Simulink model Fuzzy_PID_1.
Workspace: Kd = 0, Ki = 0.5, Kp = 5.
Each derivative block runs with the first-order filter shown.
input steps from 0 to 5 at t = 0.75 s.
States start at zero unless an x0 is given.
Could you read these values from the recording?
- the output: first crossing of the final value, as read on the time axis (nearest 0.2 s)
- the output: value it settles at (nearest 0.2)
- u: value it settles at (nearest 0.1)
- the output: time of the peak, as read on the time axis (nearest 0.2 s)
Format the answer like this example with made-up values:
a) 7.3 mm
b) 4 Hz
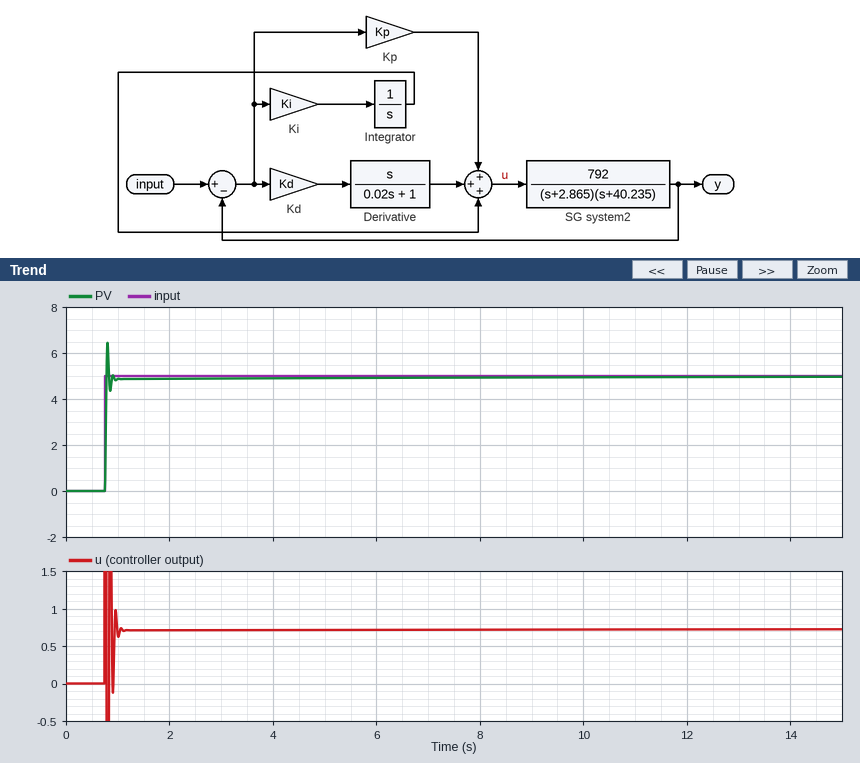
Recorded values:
a) 0.8 s
b) 5.0
c) 0.7
d) 0.8 s
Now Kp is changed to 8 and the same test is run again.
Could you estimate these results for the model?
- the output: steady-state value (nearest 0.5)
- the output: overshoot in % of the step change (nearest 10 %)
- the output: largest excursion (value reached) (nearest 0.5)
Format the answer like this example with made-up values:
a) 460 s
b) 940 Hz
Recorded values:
a) 5.0
b) 40 %
c) 7.0
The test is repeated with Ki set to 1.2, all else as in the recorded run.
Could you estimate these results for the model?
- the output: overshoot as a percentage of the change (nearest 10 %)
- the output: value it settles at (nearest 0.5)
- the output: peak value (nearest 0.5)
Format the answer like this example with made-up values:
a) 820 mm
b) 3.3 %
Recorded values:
a) 30 %
b) 5.0
c) 6.5
